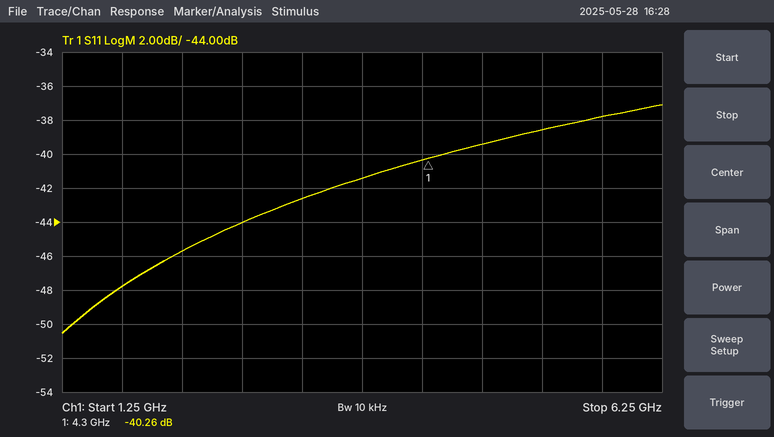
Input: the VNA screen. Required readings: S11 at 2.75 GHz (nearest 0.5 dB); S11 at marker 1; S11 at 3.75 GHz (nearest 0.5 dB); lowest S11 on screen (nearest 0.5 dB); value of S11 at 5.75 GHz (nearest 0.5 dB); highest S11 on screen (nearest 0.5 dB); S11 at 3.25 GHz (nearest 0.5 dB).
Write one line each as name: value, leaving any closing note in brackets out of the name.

S11 at 2.75 GHz: -44.0 dB
S11 at marker 1: -40.26 dB
S11 at 3.75 GHz: -41.5 dB
lowest S11 on screen: -50.5 dB
value of S11 at 5.75 GHz: -38.0 dB
highest S11 on screen: -37.0 dB
S11 at 3.25 GHz: -42.5 dB
